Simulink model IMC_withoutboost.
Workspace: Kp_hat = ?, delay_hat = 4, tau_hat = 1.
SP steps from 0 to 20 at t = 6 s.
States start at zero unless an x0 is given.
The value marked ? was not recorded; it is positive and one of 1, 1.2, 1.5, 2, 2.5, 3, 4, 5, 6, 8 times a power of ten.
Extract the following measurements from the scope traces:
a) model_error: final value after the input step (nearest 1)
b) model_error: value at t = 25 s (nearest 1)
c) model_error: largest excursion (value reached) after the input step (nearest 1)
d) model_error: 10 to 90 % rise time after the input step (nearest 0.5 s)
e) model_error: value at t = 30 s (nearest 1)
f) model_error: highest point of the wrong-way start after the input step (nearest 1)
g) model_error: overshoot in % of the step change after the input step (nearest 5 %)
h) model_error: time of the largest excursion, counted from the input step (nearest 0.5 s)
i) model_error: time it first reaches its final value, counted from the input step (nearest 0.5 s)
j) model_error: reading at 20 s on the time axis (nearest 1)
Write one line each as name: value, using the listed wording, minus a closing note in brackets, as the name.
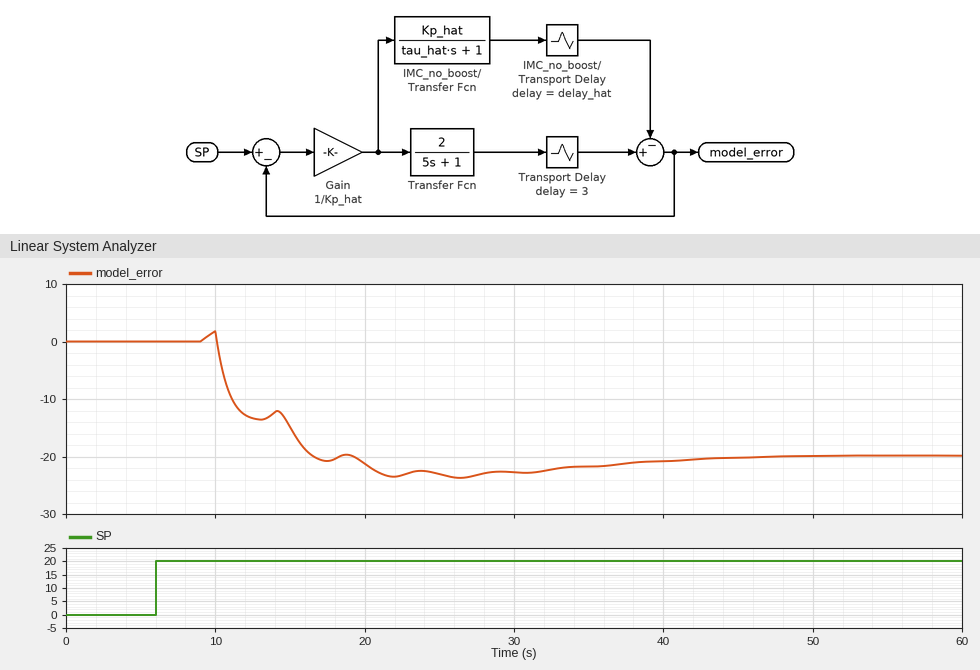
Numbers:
model_error: final value after the input step: -20
model_error: value at t = 25 s: -23
model_error: largest excursion (value reached) after the input step: -24
model_error: 10 to 90 % rise time after the input step: 5.5 s
model_error: value at t = 30 s: -23
model_error: highest point of the wrong-way start after the input step: 2
model_error: overshoot in % of the step change after the input step: 20 %
model_error: time of the largest excursion, counted from the input step: 20.5 s
model_error: time it first reaches its final value, counted from the input step: 10.5 s
model_error: reading at 20 s on the time axis: -21
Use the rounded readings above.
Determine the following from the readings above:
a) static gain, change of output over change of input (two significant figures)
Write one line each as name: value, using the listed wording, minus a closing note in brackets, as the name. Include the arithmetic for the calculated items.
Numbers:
static gain, change of output over change of input: (-20 - 0) / (20 - 0) = -1.0
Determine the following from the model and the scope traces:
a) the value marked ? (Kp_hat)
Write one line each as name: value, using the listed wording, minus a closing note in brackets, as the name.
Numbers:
the value marked ?: 4
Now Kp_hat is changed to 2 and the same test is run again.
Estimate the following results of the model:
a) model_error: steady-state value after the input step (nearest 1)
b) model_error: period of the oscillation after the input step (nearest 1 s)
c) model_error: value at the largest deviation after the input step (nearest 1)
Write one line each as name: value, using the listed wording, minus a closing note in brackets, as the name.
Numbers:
model_error: steady-state value after the input step: 0
model_error: period of the oscillation after the input step: 4 s
model_error: value at the largest deviation after the input step: -8
